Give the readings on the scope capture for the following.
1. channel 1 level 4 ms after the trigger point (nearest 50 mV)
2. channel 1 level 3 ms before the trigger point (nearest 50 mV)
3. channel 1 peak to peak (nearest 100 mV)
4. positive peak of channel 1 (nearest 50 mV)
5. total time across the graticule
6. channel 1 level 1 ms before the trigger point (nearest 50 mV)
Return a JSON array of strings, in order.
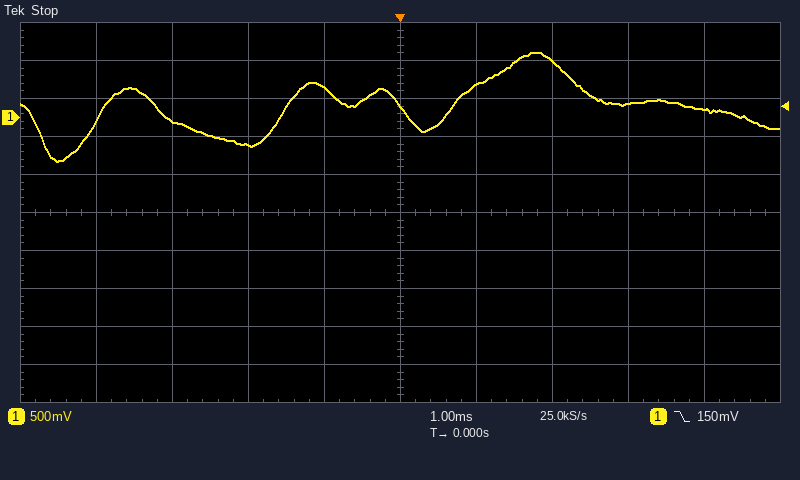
["100 mV", "-50 mV", "1.40 V", "850 mV", "10 ms", "400 mV"]
